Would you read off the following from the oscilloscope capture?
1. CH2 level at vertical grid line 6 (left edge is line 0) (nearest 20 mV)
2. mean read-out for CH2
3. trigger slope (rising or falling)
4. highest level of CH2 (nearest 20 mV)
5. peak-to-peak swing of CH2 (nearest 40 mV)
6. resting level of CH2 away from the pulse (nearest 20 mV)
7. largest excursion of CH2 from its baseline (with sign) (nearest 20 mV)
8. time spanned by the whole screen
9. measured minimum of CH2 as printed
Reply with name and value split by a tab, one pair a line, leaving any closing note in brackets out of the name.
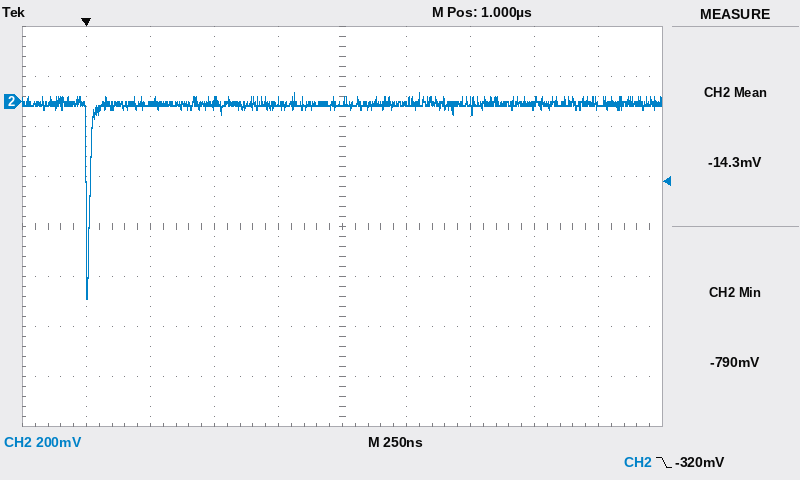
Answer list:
CH2 level at vertical grid line 6 (left edge is line 0)	0 mV
mean read-out for CH2	-14.3 mV
trigger slope	falling
highest level of CH2	40 mV
peak-to-peak swing of CH2	840 mV
resting level of CH2 away from the pulse	0 mV
largest excursion of CH2 from its baseline (with sign)	-780 mV
time spanned by the whole screen	2.5 µs
measured minimum of CH2 as printed	-790 mV
